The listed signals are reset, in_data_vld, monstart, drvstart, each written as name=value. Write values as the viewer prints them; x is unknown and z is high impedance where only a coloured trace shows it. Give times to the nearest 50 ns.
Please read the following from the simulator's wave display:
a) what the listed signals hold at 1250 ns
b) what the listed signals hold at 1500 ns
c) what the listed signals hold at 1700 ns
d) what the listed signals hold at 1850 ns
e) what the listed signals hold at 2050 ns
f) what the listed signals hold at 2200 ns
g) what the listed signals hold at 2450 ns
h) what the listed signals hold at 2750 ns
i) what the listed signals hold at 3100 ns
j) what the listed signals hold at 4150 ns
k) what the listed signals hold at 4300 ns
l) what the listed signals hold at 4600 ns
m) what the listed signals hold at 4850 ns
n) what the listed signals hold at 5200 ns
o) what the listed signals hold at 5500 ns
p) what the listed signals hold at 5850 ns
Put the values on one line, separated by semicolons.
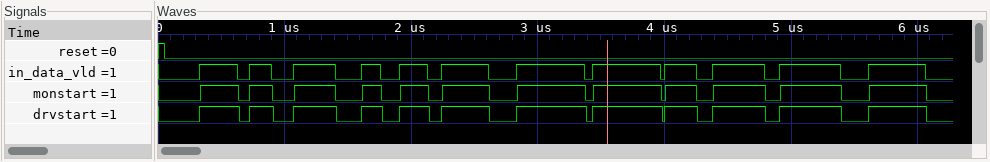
reset=0, in_data_vld=1, monstart=1, drvstart=1; reset=0, in_data_vld=0, monstart=0, drvstart=0; reset=0, in_data_vld=1, monstart=1, drvstart=1; reset=0, in_data_vld=0, monstart=0, drvstart=0; reset=0, in_data_vld=1, monstart=1, drvstart=1; reset=0, in_data_vld=0, monstart=0, drvstart=0; reset=0, in_data_vld=1, monstart=1, drvstart=1; reset=0, in_data_vld=0, monstart=0, drvstart=0; reset=0, in_data_vld=1, monstart=1, drvstart=1; reset=0, in_data_vld=1, monstart=1, drvstart=1; reset=0, in_data_vld=0, monstart=0, drvstart=0; reset=0, in_data_vld=1, monstart=1, drvstart=1; reset=0, in_data_vld=0, monstart=0, drvstart=0; reset=0, in_data_vld=1, monstart=1, drvstart=1; reset=0, in_data_vld=0, monstart=0, drvstart=0; reset=0, in_data_vld=1, monstart=1, drvstart=1
